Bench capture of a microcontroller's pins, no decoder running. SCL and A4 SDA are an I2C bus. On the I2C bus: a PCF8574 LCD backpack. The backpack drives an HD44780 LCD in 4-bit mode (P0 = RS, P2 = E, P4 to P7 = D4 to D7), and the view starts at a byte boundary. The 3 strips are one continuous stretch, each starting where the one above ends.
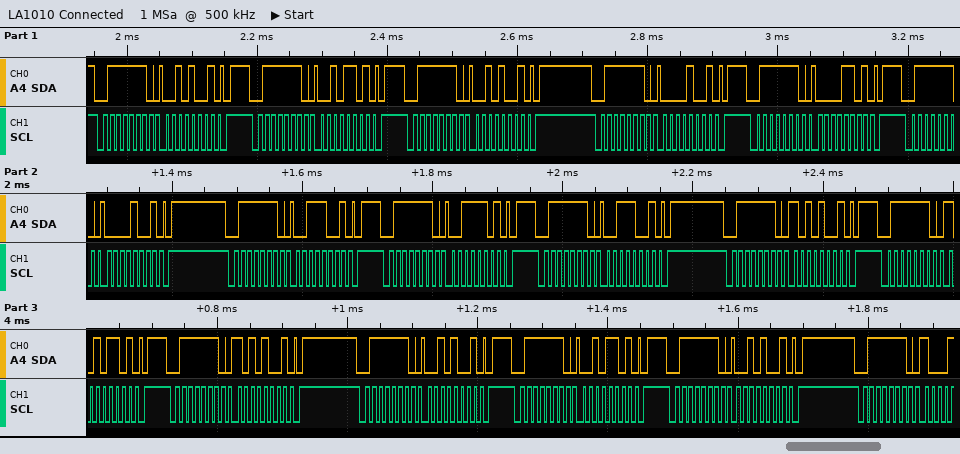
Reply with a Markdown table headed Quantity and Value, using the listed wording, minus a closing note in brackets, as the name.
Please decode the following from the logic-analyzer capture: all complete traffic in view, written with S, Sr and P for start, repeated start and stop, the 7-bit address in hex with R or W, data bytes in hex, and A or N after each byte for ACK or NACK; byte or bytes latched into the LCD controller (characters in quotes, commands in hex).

| Quantity | Value |
|---|---|
| all complete traffic in view, written with S, Sr and P for start, repeated start and stop, the 7-bit address in hex with R or W, data bytes in hex, and A or N after each byte for ACK or NACK | S 3FW A 29 A P S 3FW A 2D A P S 3FW A 29 A P S 3FW A 09 A P S 3FW A 0D A P S 3FW A 09 A P S 3FW A 39 A P S 3FW A 3D A P S 3FW A 39 A P S 3FW A A9 A P S 3FW A AD A P S 3FW A A9 A P S 3FW A 29 A P S 3FW A 2D A P S 3FW A 29 A P S 3FW A |
| byte or bytes latched into the LCD controller | ' ' ':' |
